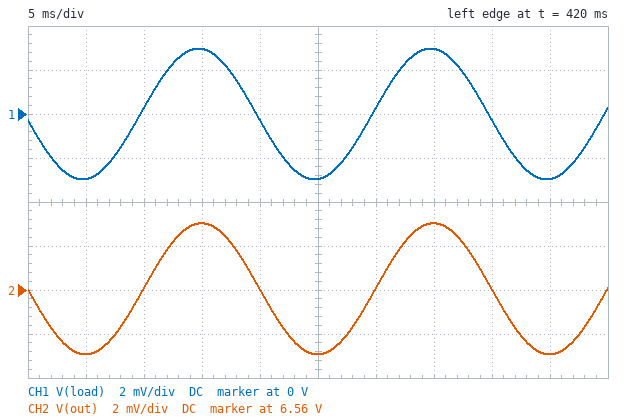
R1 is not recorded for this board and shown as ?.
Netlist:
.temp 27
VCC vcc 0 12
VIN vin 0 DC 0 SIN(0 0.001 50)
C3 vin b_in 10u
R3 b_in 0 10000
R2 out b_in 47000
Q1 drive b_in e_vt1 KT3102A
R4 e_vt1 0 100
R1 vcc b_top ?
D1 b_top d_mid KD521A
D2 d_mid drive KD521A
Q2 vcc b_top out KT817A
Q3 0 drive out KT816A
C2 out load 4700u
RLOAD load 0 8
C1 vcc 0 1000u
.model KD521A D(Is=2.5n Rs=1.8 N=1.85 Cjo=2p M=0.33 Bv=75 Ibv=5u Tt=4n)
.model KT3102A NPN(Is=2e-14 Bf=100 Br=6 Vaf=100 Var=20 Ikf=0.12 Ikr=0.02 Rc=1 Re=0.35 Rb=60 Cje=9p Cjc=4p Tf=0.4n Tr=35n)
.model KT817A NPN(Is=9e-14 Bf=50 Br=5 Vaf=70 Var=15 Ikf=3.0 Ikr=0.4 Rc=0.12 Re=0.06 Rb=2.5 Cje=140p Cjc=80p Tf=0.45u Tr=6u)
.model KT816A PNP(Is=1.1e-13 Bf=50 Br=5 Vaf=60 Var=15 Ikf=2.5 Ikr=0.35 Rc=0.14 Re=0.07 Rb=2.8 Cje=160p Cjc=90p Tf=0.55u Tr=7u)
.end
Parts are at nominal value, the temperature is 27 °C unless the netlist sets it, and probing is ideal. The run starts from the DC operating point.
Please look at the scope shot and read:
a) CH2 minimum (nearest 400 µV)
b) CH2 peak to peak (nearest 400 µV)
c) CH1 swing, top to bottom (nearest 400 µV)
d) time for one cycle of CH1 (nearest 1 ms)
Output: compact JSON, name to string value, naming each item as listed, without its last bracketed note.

{"CH2 minimum": "6.5572 V", "CH2 peak to peak": "6.0 mV", "CH1 swing, top to bottom": "6.0 mV", "time for one cycle of CH1": "20 ms"}
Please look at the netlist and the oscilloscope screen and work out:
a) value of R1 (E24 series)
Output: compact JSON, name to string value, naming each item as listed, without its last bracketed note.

{"value of R1": "1.8 kΩ"}
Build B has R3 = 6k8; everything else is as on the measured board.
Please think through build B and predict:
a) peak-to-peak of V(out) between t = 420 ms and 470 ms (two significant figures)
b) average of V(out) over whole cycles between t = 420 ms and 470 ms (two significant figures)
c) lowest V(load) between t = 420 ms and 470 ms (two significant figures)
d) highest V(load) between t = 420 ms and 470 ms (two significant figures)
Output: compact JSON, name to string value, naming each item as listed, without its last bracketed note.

{"peak-to-peak of V(out) between t = 420 ms and 470 ms": "5.8 mV", "average of V(out) over whole cycles between t = 420 ms and 470 ms": "7.7 V", "lowest V(load) between t = 420 ms and 470 ms": "-2.9 mV", "highest V(load) between t = 420 ms and 470 ms": "2.9 mV"}
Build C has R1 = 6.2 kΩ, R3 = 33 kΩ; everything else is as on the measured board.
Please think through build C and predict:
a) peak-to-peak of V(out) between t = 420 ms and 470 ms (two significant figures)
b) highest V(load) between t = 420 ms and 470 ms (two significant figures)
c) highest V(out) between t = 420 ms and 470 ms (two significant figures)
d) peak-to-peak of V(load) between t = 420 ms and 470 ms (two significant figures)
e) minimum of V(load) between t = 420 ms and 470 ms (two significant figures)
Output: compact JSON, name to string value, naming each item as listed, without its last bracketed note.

{"peak-to-peak of V(out) between t = 420 ms and 470 ms": "6.4 mV", "highest V(load) between t = 420 ms and 470 ms": "3.2 mV", "highest V(out) between t = 420 ms and 470 ms": "2.6 V", "peak-to-peak of V(load) between t = 420 ms and 470 ms": "6.3 mV", "minimum of V(load) between t = 420 ms and 470 ms": "-3.2 mV"}
